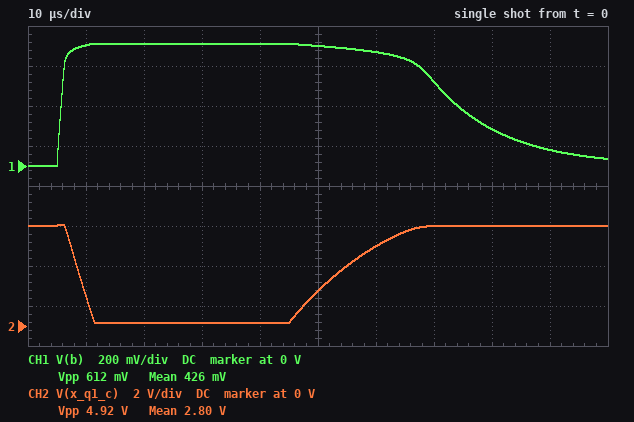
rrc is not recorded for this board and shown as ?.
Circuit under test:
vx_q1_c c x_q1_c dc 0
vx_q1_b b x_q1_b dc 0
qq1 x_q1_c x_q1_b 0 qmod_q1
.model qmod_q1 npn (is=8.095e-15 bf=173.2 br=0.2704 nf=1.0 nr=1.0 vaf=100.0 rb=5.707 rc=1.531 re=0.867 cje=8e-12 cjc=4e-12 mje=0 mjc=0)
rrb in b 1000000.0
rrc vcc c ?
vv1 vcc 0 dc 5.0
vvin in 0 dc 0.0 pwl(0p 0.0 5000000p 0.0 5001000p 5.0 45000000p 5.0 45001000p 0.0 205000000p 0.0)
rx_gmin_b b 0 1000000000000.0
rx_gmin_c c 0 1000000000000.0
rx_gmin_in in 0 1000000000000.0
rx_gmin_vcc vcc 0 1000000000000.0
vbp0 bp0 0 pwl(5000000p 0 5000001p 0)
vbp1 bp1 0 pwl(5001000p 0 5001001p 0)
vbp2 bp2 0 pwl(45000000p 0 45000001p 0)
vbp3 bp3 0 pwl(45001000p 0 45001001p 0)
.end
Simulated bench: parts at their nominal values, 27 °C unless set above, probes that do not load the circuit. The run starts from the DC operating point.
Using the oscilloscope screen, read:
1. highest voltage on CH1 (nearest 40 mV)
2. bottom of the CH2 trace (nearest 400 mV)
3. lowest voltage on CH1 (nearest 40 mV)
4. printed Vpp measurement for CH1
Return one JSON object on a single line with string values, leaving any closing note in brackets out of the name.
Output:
{"highest voltage on CH1": "600 mV", "bottom of the CH2 trace": "0 V", "lowest voltage on CH1": "0 V", "printed Vpp measurement for CH1": "612 mV"}
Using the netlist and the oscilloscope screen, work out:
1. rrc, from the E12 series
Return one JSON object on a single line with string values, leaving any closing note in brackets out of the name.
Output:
{"rrc, from the E12 series": "33 kΩ"}
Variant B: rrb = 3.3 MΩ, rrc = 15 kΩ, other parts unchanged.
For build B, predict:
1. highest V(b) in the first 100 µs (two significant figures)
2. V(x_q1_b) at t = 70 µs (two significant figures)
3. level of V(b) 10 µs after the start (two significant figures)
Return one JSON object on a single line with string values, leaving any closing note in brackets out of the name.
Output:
{"highest V(b) in the first 100 µs": "620 mV", "V(x_q1_b) at t = 70 µs": "520 mV", "level of V(b) 10 µs after the start": "540 mV"}
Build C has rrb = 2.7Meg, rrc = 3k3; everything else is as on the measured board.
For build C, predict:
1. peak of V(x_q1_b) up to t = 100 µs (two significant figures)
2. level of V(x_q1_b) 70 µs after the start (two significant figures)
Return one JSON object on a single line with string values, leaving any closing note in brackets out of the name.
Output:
{"peak of V(x_q1_b) up to t = 100 µs": "630 mV", "level of V(x_q1_b) 70 µs after the start": "310 mV"}
